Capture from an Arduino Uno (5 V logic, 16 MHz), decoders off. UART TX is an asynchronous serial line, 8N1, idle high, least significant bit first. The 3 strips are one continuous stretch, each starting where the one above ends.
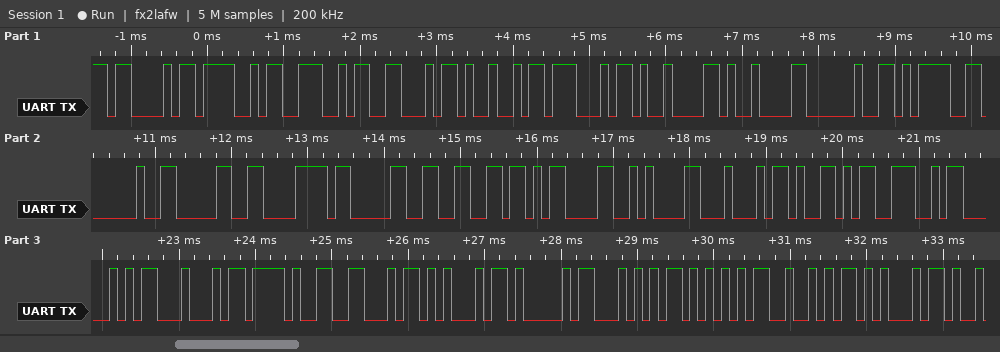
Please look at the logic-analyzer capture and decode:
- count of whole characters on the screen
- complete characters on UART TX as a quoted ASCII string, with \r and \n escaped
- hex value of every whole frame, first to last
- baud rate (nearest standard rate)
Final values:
30
"CONFIG\t\t = 0x0f\r\nDYNPD/FEATURE"
0x43 0x4F 0x4E 0x46 0x49 0x47 0x09 0x09 0x20 0x3D 0x20 0x30 0x78 0x30 0x66 0x0D 0x0A 0x44 0x59 0x4E 0x50 0x44 0x2F 0x46 0x45 0x41 0x54 0x55 0x52 0x45
9600 baud
